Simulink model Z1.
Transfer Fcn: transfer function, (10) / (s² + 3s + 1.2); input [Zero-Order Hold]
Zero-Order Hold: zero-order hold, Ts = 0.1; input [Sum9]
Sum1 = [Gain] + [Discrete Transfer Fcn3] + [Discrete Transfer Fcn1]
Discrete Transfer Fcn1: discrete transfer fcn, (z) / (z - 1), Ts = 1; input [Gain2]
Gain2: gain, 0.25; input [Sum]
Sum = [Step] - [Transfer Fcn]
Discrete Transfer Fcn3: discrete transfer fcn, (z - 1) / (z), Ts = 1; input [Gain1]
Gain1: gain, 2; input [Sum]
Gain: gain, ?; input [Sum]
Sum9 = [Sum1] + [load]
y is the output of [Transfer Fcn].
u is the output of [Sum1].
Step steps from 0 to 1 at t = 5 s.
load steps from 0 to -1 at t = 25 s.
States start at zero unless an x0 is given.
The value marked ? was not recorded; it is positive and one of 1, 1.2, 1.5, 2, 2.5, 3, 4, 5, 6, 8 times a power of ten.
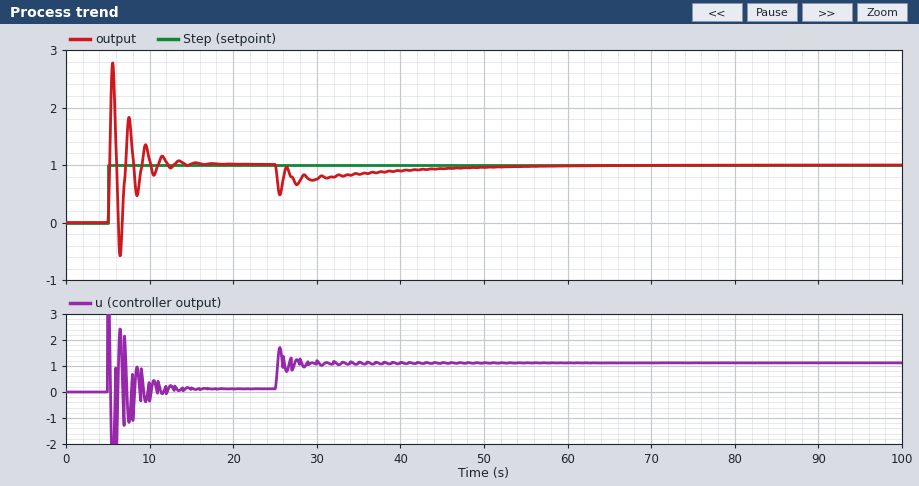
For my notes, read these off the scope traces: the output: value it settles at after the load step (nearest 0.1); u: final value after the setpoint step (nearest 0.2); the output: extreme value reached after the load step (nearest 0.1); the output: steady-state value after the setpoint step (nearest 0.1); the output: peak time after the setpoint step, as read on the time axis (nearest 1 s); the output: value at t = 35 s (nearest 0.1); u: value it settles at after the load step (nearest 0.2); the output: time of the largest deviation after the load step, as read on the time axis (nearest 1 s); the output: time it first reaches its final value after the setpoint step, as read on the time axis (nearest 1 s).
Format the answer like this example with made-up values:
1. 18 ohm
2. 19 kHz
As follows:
1. 1.0
2. 0.2
3. 0.5
4. 1.0
5. 6 s
6. 0.8
7. 1.2
8. 26 s
9. 5 s
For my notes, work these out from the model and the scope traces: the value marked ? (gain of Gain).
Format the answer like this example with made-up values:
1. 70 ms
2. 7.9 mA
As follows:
1. 3
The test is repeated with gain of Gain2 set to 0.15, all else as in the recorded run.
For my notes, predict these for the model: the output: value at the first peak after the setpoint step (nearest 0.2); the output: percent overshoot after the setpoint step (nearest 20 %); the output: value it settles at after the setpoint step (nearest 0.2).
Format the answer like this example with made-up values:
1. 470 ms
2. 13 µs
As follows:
1. 2.8
2. 180 %
3. 1.0
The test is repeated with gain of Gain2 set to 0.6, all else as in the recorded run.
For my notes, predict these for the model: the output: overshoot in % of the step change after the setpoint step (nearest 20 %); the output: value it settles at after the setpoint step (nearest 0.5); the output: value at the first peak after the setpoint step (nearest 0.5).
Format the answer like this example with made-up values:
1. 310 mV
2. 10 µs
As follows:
1. 200 %
2. 1.0
3. 3.0
